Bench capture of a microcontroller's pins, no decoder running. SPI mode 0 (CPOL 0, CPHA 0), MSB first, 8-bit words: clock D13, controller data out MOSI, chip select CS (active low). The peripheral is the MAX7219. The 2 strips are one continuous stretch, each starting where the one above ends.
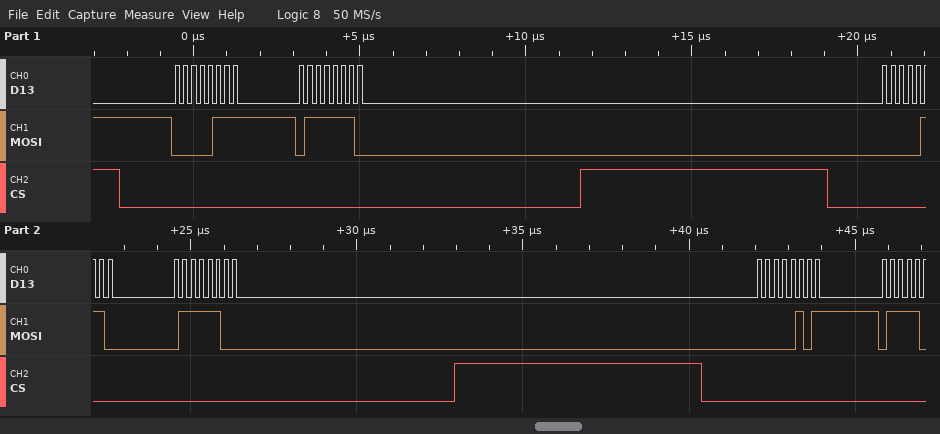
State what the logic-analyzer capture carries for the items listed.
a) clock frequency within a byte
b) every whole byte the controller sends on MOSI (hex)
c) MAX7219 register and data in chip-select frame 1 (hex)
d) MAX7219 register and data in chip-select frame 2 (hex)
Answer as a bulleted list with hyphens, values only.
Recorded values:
- 4 MHz
- 0x07 0x7E 0x06 0x7C 0x05
- register 0x7, data 0x7E
- register 0x6, data 0x7C
